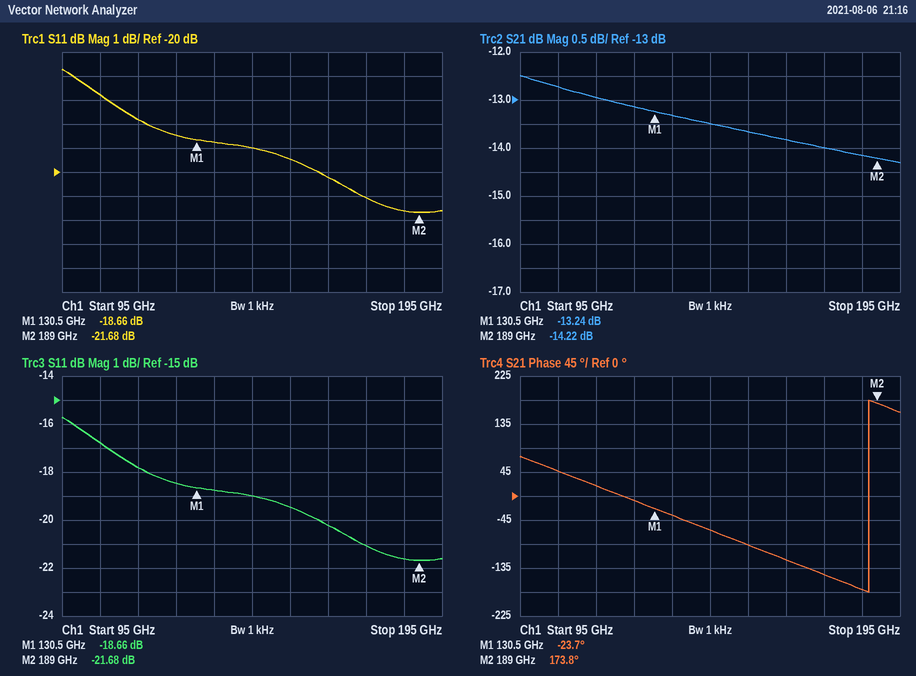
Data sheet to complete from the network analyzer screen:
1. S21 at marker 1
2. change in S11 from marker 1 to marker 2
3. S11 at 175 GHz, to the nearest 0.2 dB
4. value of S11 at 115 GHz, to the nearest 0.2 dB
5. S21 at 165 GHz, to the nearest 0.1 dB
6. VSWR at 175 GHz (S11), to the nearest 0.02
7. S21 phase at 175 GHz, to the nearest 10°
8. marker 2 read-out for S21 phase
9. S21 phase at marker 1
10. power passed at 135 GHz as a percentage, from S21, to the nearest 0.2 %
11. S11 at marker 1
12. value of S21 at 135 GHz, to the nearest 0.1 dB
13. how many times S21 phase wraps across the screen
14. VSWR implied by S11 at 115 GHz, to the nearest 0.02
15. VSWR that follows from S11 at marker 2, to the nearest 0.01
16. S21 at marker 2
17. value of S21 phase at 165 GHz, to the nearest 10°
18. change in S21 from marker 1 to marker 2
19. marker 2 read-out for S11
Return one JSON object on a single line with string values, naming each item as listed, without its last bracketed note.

{"S21 at marker 1": "-13.24 dB", "change in S11 from marker 1 to marker 2": "-3.02 dB", "S11 at 175 GHz, to the nearest 0.2 dB": "-21.0 dB", "value of S11 at 115 GHz, to the nearest 0.2 dB": "-17.8 dB", "S21 at 165 GHz, to the nearest 0.1 dB": "-13.8 dB", "VSWR at 175 GHz (S11), to the nearest 0.02": "1.20", "S21 phase at 175 GHz, to the nearest 10°": "-150°", "marker 2 read-out for S21 phase": "173.8°", "S21 phase at marker 1": "-23.7°", "power passed at 135 GHz as a percentage, from S21, to the nearest 0.2 %": "4.6 %", "S11 at marker 1": "-18.66 dB", "value of S21 at 135 GHz, to the nearest 0.1 dB": "-13.3 dB", "how many times S21 phase wraps across the screen": "1", "VSWR implied by S11 at 115 GHz, to the nearest 0.02": "1.30", "VSWR that follows from S11 at marker 2, to the nearest 0.01": "1.18", "S21 at marker 2": "-14.22 dB", "value of S21 phase at 165 GHz, to the nearest 10°": "-120°", "change in S21 from marker 1 to marker 2": "-0.98 dB", "marker 2 read-out for S11": "-21.68 dB"}
